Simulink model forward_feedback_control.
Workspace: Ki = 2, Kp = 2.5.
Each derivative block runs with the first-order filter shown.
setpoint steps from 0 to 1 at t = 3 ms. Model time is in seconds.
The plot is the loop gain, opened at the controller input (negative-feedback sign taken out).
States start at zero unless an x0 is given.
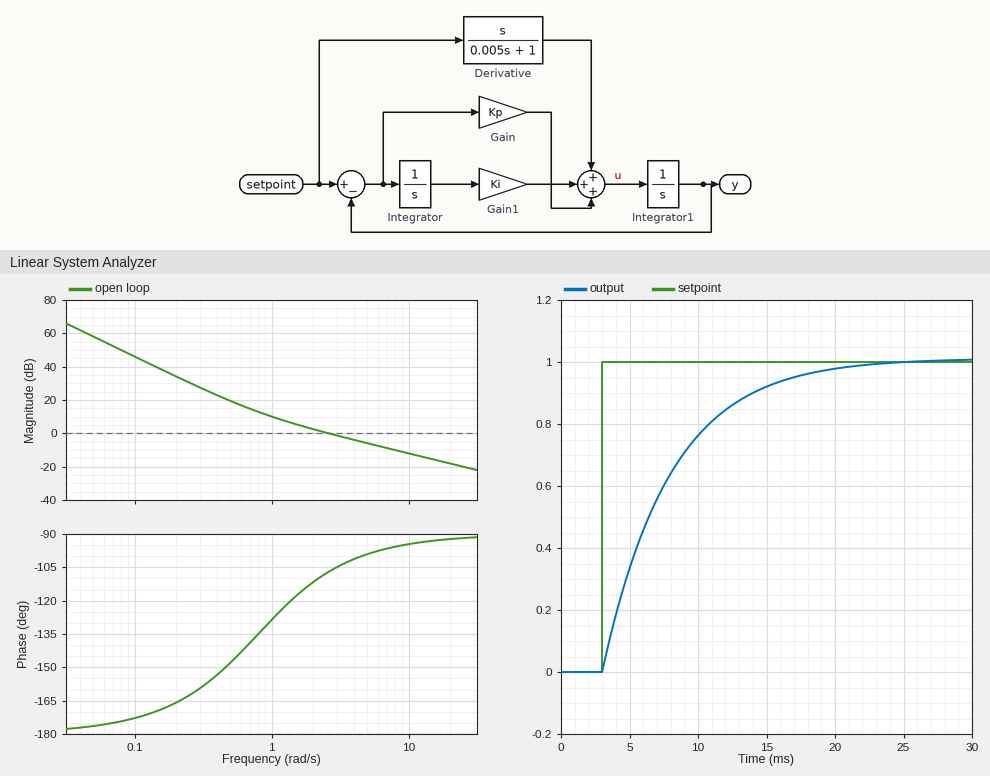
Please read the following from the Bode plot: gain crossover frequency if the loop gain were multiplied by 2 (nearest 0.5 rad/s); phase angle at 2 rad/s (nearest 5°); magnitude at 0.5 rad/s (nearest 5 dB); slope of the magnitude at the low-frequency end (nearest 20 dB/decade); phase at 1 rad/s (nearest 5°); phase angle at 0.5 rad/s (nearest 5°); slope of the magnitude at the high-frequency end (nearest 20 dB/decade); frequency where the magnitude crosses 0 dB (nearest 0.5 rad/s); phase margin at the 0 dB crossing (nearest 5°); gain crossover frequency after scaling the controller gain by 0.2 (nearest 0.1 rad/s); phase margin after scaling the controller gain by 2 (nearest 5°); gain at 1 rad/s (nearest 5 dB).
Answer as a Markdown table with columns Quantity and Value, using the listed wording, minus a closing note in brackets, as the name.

| Quantity | Value |
|---|---|
| gain crossover frequency if the loop gain were multiplied by 2 | 5.0 rad/s |
| phase angle at 2 rad/s | -110° |
| magnitude at 0.5 rad/s | 20 dB |
| slope of the magnitude at the low-frequency end | -40 dB/decade |
| phase at 1 rad/s | -130° |
| phase angle at 0.5 rad/s | -150° |
| slope of the magnitude at the high-frequency end | -20 dB/decade |
| frequency where the magnitude crosses 0 dB | 2.5 rad/s |
| phase margin at the 0 dB crossing | 75° |
| gain crossover frequency after scaling the controller gain by 0.2 | 0.7 rad/s |
| phase margin after scaling the controller gain by 2 | 80° |
| gain at 1 rad/s | 10 dB |
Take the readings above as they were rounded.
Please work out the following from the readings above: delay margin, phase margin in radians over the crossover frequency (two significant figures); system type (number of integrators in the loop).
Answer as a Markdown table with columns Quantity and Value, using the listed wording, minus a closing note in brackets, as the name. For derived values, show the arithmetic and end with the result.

| Quantity | Value |
|---|---|
| delay margin, phase margin in radians over the crossover frequency | 75 × π / 180 / 2.5 = 0.52 s |
| system type | 2 |
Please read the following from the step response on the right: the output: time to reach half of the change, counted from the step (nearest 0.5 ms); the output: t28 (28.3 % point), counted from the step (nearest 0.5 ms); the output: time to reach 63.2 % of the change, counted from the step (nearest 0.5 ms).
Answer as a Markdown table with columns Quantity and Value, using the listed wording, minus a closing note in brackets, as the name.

| Quantity | Value |
|---|---|
| the output: time to reach half of the change, counted from the step | 3.5 ms |
| the output: t28 (28.3 % point), counted from the step | 1.5 ms |
| the output: time to reach 63.2 % of the change, counted from the step | 5.0 ms |
